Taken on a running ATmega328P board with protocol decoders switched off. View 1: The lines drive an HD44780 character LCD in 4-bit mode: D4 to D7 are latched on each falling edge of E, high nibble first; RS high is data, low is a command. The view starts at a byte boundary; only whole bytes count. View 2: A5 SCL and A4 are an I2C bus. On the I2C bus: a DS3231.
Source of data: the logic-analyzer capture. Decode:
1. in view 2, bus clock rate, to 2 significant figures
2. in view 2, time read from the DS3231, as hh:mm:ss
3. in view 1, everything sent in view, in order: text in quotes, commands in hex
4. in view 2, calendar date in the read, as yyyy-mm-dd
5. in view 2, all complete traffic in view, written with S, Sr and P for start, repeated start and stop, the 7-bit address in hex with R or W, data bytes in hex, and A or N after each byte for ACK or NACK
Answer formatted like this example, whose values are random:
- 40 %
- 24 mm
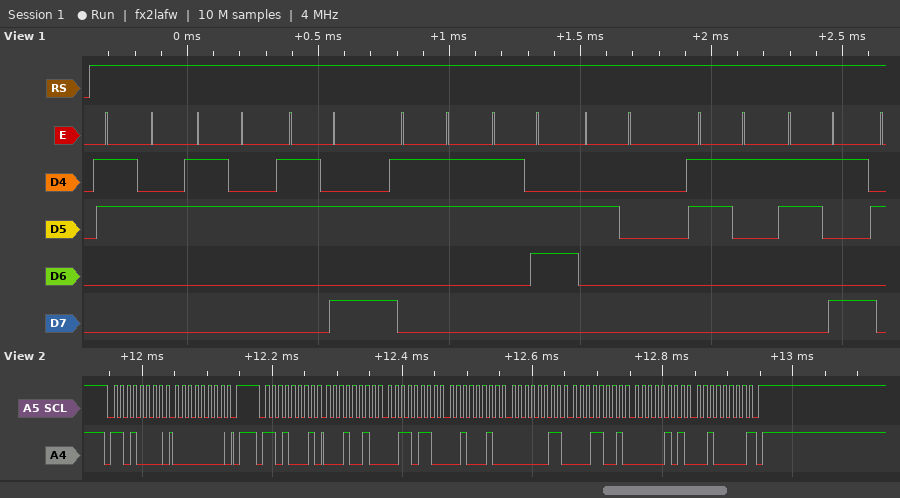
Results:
- 100 kHz
- 22:36:12
- "22:36 19"
- 2020-05-19
- S 68W A 00 A P S 68R A 12 A 36 A 22 A 03 A 19 A 05 A 20 N P
